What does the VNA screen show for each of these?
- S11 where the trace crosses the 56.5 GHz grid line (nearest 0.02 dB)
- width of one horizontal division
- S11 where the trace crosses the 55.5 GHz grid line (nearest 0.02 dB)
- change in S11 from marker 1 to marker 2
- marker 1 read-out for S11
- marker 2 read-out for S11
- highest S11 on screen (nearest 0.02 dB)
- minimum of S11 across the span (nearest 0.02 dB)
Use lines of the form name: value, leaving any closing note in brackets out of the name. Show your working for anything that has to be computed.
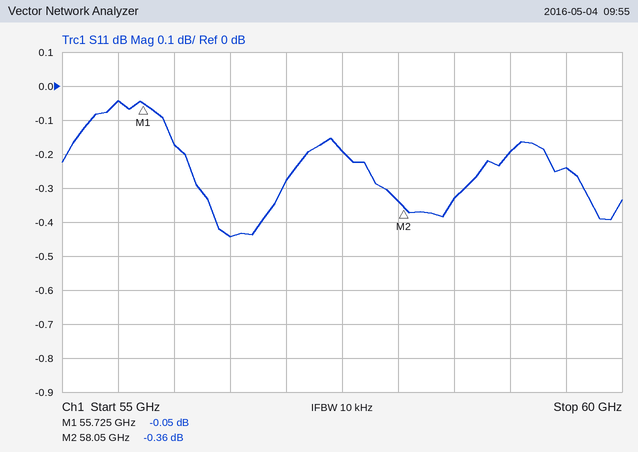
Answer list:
S11 where the trace crosses the 56.5 GHz grid line: -0.44 dB
width of one horizontal division: 500 MHz
S11 where the trace crosses the 55.5 GHz grid line: -0.04 dB
change in S11 from marker 1 to marker 2: -0.36 − (-0.05) = -0.31 dB
marker 1 read-out for S11: -0.05 dB
marker 2 read-out for S11: -0.36 dB
highest S11 on screen: -0.04 dB
minimum of S11 across the span: -0.44 dB
